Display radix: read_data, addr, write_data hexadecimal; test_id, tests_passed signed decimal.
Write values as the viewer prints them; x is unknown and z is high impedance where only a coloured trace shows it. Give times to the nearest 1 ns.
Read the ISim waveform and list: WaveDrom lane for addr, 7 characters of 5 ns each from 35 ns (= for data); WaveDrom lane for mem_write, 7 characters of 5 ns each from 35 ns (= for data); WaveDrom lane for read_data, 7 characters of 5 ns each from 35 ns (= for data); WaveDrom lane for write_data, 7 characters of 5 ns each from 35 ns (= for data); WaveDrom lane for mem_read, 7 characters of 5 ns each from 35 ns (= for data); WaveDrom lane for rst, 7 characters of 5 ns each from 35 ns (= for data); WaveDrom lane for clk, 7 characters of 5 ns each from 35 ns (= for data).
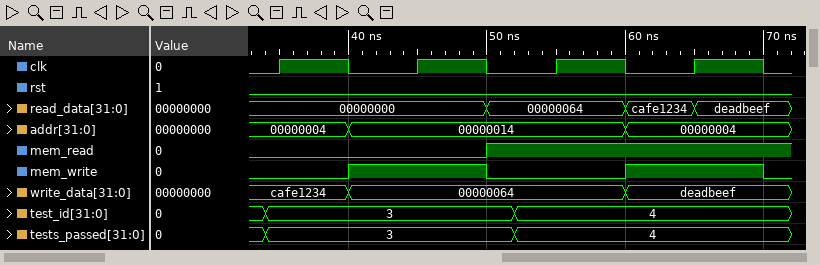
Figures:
{name: 'addr', wave: '==...=.', data: '00000004 00000014 00000004'}
{name: 'mem_write', wave: '01.0.1.'}
{name: 'read_data', wave: '=..=.==', data: '00000000 00000064 cafe1234 deadbeef'}
{name: 'write_data', wave: '==...=.', data: 'cafe1234 00000064 deadbeef'}
{name: 'mem_read', wave: '0..1...'}
{name: 'rst', wave: '0......'}
{name: 'clk', wave: '1010101'}
